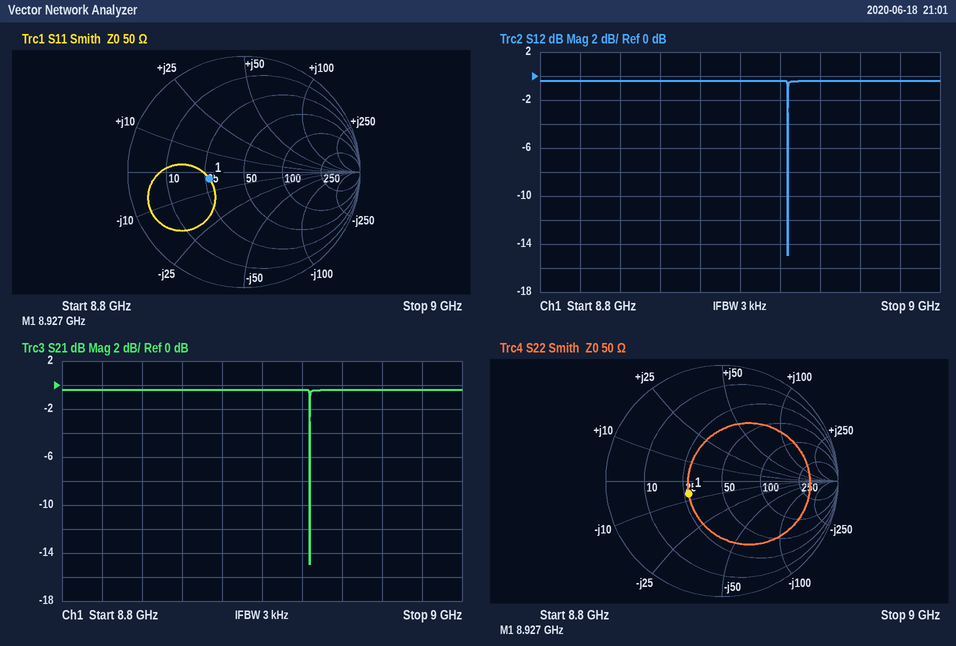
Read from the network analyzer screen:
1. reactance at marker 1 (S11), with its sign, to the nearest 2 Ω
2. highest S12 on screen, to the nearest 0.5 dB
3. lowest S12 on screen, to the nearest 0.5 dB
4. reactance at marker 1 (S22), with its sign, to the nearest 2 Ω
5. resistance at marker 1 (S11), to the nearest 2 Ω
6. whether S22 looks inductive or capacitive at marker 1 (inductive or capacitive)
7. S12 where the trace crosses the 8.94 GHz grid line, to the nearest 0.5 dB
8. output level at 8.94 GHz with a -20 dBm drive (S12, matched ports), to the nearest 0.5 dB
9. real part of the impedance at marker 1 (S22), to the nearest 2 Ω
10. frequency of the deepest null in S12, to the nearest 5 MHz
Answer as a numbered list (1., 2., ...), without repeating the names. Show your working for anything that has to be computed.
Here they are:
1. -4 Ω
2. -0.5 dB
3. -15.0 dB
4. -6 Ω
5. 26 Ω
6. capacitive
7. -0.5 dB
8. -20 dBm + (-0.5 dB) = -20.5 dBm
9. 28 Ω
10. 8.925 GHz
